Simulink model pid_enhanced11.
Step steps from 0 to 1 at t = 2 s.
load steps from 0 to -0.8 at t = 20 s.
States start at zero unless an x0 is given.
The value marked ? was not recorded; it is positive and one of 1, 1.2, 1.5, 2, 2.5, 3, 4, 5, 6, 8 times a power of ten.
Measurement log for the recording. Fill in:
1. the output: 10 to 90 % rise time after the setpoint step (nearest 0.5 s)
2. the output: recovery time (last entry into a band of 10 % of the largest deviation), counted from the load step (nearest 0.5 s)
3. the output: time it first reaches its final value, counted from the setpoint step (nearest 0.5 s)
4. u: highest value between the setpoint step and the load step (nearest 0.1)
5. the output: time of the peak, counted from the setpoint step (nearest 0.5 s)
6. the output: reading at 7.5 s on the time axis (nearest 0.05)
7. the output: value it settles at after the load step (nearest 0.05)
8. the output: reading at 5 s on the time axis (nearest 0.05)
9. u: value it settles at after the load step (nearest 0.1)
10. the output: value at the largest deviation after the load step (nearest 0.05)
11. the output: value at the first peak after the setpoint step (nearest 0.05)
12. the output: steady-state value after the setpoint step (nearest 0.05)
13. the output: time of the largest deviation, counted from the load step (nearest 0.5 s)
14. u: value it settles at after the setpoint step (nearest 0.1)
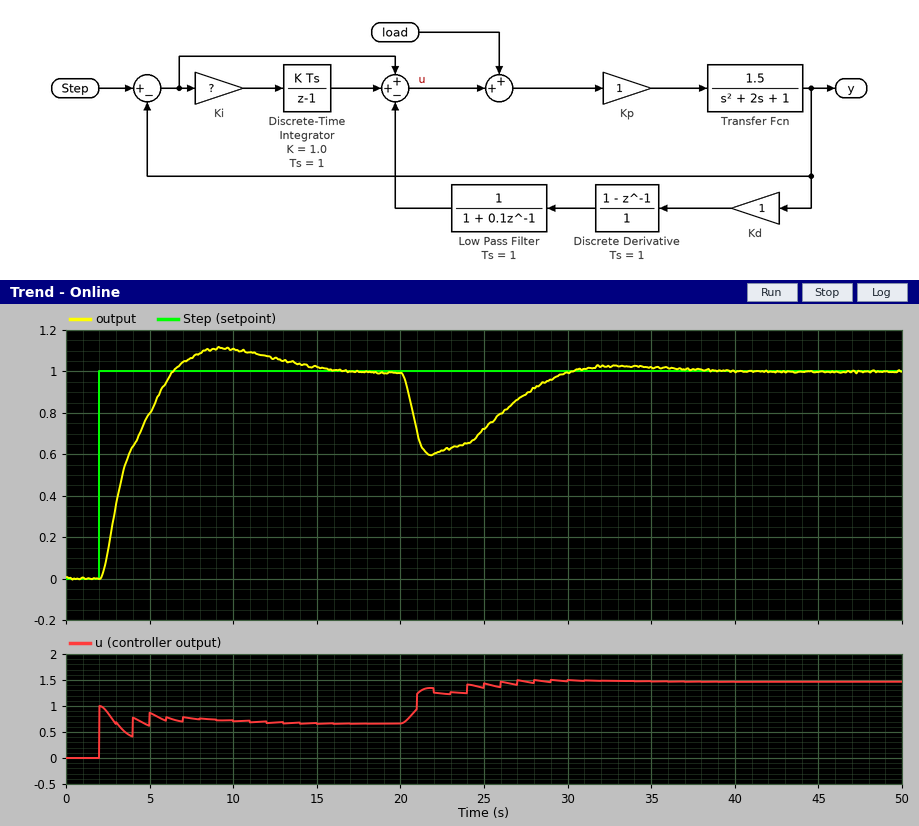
3.0 s
9.0 s
4.5 s
1.0
7.5 s
1.05
1.00
0.80
1.5
0.60
1.10
1.00
2.0 s
0.7
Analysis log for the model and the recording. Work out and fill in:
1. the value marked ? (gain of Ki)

0.4
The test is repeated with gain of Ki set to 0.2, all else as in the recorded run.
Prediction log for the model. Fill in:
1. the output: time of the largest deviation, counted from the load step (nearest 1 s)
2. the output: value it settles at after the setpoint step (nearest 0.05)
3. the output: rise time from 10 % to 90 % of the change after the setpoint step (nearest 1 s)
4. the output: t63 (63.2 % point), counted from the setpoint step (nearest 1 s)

4 s
1.00
6 s
3 s
